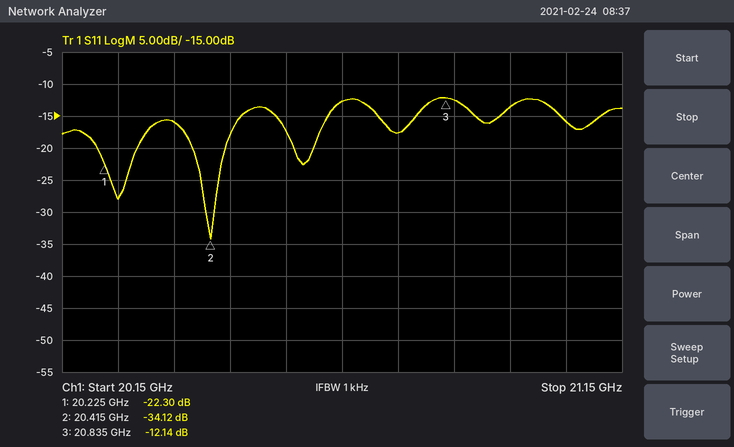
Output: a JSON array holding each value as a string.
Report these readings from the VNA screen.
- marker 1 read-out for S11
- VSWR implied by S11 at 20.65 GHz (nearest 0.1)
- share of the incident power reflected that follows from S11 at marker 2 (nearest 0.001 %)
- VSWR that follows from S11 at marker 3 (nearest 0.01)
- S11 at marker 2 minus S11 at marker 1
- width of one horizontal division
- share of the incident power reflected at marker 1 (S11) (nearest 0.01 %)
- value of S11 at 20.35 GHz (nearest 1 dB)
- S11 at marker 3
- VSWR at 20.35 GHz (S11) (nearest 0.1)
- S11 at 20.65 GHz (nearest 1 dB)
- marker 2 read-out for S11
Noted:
["-22.30 dB", "1.6", "0.039 %", "1.66", "-11.82 dB", "100 MHz", "0.59 %", "-16 dB", "-12.14 dB", "1.4", "-13 dB", "-34.12 dB"]
